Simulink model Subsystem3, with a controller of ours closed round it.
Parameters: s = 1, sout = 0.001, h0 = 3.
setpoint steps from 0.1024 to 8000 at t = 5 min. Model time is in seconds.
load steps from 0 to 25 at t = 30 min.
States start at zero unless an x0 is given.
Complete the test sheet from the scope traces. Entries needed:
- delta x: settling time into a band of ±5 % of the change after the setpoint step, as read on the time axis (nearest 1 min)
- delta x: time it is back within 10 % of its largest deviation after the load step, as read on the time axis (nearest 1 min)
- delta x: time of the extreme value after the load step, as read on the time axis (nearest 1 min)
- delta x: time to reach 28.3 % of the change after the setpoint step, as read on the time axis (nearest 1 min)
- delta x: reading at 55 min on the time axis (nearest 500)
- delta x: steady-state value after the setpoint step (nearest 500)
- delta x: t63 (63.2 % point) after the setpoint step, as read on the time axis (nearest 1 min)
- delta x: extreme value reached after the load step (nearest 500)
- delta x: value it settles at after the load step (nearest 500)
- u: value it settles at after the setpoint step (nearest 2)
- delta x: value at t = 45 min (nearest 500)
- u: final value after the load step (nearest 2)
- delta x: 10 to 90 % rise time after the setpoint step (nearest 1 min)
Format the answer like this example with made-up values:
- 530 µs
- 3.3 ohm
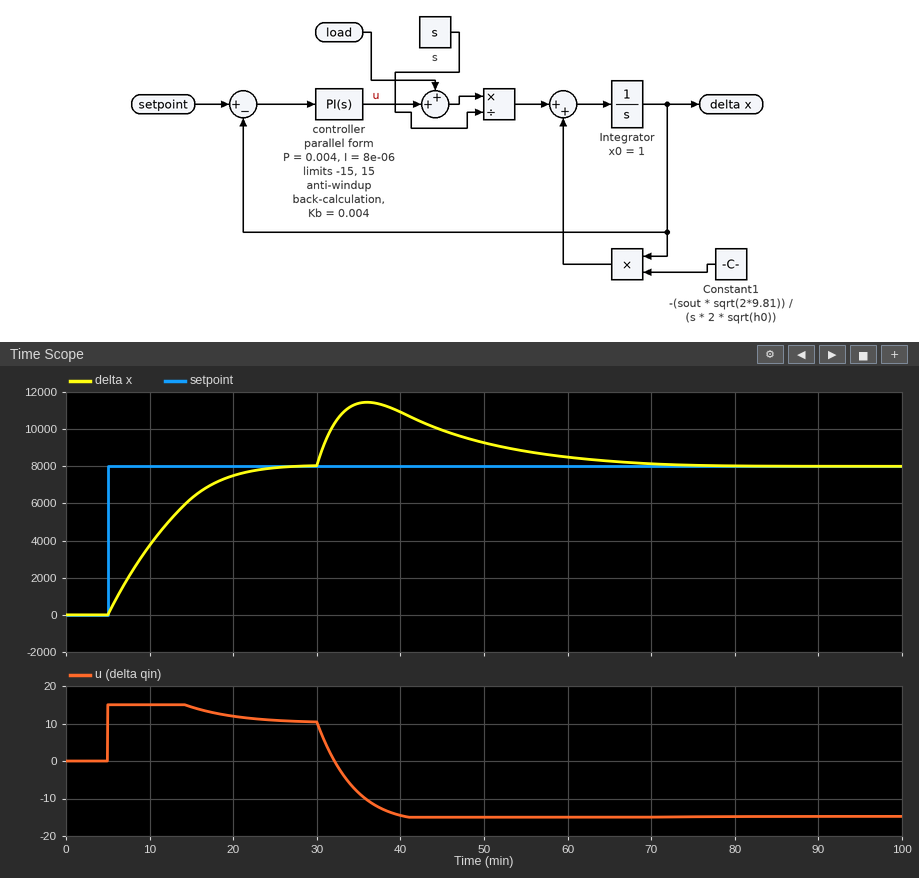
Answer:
- 21 min
- 63 min
- 36 min
- 8 min
- 9000
- 8000
- 12 min
- 11500
- 8000
- 10
- 10000
- -14
- 12 min
